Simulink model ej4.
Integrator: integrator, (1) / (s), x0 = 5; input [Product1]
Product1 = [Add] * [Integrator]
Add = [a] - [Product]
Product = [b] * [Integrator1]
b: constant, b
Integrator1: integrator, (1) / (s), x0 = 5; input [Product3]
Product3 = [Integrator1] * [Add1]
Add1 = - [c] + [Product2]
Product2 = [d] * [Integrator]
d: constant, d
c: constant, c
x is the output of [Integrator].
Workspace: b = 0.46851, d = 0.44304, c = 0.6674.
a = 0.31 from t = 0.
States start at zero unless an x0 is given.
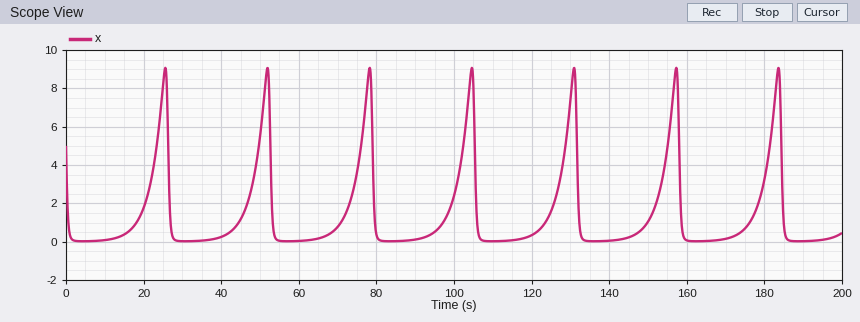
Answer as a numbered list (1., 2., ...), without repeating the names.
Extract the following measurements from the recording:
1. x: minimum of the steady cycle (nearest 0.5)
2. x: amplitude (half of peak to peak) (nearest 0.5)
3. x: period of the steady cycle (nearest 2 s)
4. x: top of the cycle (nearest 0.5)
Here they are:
1. 0.0
2. 4.5
3. 26 s
4. 9.0
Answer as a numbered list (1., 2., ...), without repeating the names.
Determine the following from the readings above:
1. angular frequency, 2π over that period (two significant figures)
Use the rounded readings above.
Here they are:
1. 0.24 rad/s
